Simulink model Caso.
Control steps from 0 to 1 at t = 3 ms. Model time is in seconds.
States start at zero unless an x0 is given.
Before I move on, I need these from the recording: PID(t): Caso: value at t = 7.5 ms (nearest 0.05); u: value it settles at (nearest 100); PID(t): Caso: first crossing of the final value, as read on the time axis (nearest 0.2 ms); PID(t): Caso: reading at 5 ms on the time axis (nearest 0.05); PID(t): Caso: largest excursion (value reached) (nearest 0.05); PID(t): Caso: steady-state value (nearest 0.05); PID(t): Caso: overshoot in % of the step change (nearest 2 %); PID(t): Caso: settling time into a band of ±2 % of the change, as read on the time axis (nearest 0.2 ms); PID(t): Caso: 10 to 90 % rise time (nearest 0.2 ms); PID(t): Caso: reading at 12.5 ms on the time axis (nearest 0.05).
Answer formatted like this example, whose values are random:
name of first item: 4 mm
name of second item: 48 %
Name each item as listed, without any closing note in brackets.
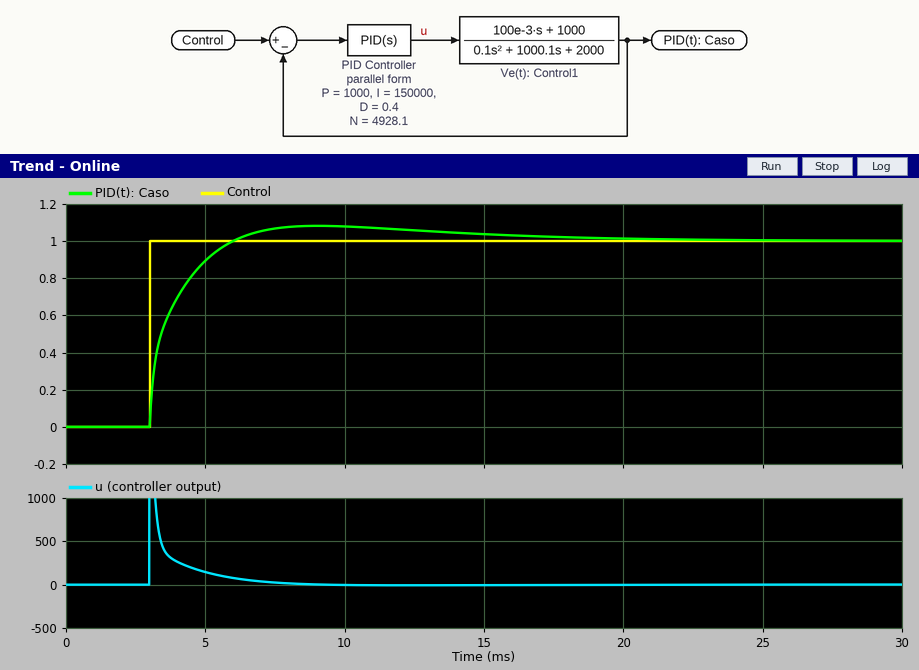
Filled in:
PID(t): Caso: value at t = 7.5 ms: 1.05
u: value it settles at: 0
PID(t): Caso: first crossing of the final value, as read on the time axis: 6.0 ms
PID(t): Caso: reading at 5 ms on the time axis: 0.90
PID(t): Caso: largest excursion (value reached): 1.10
PID(t): Caso: steady-state value: 1.00
PID(t): Caso: overshoot in % of the step change: 8 %
PID(t): Caso: settling time into a band of ±2 % of the change, as read on the time axis: 18.2 ms
PID(t): Caso: 10 to 90 % rise time: 2.0 ms
PID(t): Caso: reading at 12.5 ms on the time axis: 1.05
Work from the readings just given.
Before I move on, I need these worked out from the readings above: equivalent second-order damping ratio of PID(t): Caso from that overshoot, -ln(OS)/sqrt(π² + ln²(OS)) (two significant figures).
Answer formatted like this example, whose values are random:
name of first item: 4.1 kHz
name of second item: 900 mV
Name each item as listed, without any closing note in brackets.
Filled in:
equivalent second-order damping ratio of PID(t): Caso from that overshoot, -ln(OS)/sqrt(π² + ln²(OS)): 0.63
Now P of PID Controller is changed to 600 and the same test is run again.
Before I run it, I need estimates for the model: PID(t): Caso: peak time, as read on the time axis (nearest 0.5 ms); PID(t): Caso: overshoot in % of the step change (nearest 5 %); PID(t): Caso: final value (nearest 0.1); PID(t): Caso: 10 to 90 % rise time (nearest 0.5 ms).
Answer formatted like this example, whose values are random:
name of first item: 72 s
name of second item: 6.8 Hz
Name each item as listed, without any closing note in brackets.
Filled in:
PID(t): Caso: peak time, as read on the time axis: 10.0 ms
PID(t): Caso: overshoot in % of the step change: 15 %
PID(t): Caso: final value: 1.0
PID(t): Caso: 10 to 90 % rise time: 2.5 ms
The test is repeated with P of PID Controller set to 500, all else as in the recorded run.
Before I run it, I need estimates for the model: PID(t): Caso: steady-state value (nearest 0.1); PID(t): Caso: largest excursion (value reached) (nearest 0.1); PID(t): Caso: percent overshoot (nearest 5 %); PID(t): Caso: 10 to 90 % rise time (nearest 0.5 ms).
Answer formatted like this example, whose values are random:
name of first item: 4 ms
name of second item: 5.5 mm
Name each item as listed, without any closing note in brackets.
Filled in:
PID(t): Caso: steady-state value: 1.0
PID(t): Caso: largest excursion (value reached): 1.2
PID(t): Caso: percent overshoot: 20 %
PID(t): Caso: 10 to 90 % rise time: 3.0 ms
